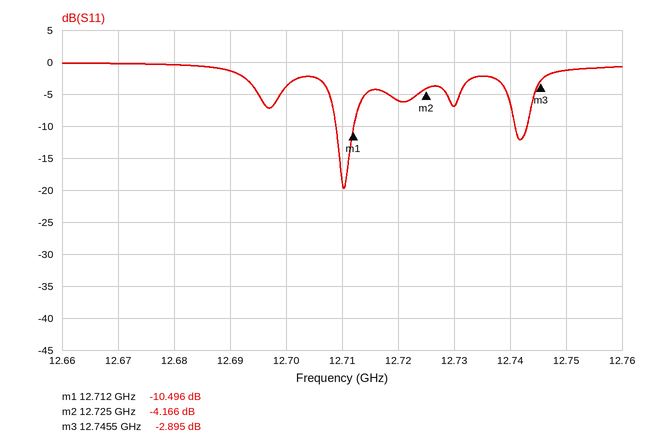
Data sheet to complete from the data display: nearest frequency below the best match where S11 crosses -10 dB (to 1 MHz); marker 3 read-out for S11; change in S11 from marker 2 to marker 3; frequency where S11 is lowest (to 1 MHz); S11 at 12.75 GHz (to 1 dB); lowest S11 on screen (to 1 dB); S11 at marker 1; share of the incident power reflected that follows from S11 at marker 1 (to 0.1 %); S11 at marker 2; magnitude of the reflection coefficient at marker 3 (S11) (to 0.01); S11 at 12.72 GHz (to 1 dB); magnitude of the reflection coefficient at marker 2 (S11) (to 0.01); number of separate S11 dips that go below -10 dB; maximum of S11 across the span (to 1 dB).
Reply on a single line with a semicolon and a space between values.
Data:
12.709 GHz; -2.895 dB; 1.271 dB; 12.710 GHz; -1 dB; -20 dB; -10.496 dB; 8.9 %; -4.166 dB; 0.72; -6 dB; 0.62; 2; 0 dB
